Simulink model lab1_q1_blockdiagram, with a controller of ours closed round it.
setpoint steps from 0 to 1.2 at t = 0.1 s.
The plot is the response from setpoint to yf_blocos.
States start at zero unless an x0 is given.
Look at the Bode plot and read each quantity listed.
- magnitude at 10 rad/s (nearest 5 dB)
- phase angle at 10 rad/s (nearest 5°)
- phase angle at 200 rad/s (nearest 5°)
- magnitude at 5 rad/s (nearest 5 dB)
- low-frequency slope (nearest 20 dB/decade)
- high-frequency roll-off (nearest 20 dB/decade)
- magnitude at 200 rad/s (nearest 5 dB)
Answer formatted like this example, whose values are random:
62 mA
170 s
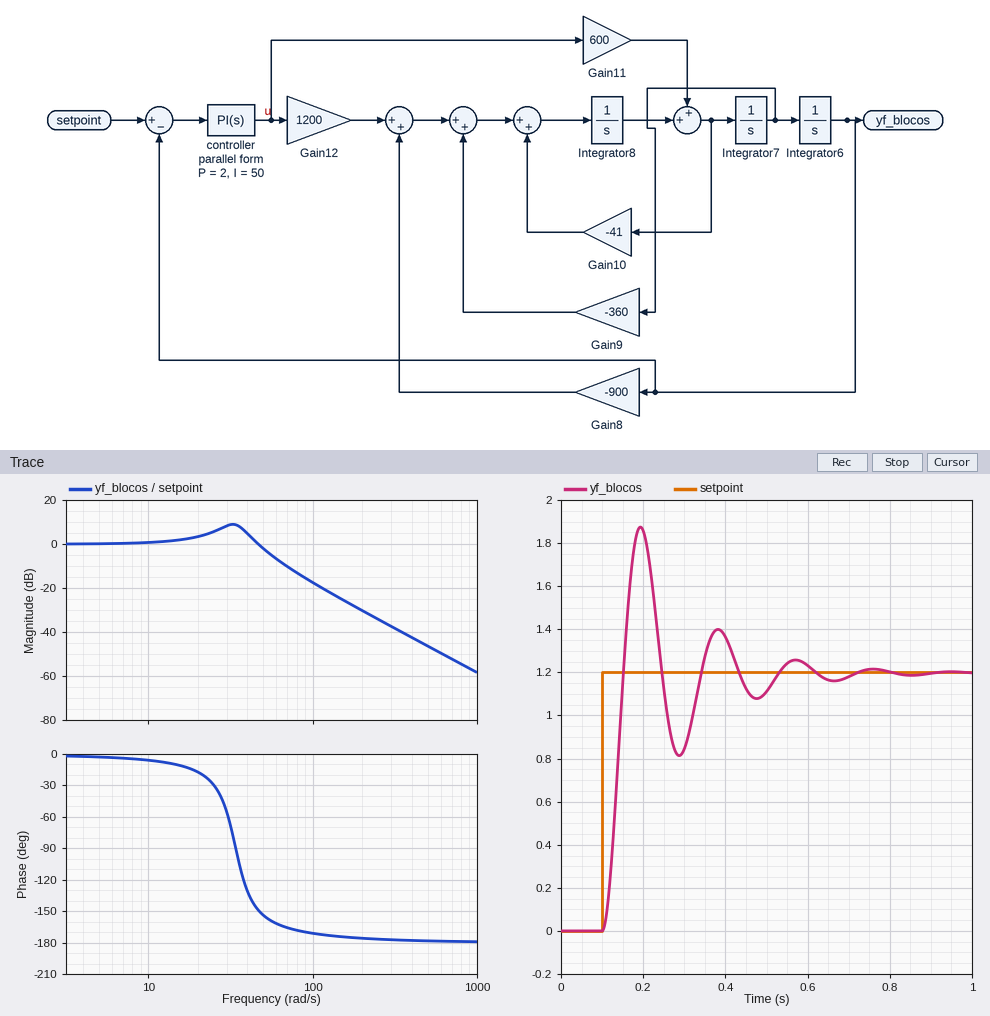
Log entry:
0 dB
-5°
-175°
0 dB
0 dB/decade
-40 dB/decade
-30 dB
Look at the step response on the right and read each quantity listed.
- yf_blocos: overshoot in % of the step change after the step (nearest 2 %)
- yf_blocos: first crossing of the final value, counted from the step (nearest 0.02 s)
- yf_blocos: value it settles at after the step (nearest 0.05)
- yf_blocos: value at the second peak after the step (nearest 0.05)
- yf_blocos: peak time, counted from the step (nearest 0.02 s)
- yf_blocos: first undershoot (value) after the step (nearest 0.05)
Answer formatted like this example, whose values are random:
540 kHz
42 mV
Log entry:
56 %
0.06 s
1.20
1.40
0.10 s
0.80
